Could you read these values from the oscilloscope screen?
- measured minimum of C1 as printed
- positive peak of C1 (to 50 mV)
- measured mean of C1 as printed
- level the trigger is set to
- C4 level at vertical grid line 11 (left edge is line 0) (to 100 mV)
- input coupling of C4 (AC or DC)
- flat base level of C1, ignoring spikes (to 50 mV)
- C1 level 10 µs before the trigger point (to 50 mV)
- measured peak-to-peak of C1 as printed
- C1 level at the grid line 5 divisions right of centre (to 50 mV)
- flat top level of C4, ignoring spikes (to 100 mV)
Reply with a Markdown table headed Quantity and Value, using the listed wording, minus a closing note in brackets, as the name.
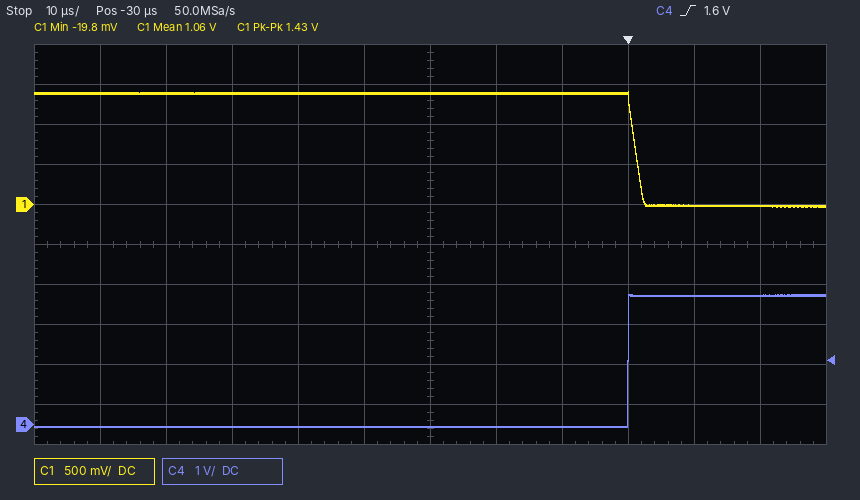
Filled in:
| Quantity | Value |
|---|---|
| measured minimum of C1 as printed | -19.8 mV |
| positive peak of C1 | 1.40 V |
| measured mean of C1 as printed | 1.06 V |
| level the trigger is set to | 1.6 V |
| C4 level at vertical grid line 11 (left edge is line 0) | 3.2 V |
| input coupling of C4 | DC |
| flat base level of C1, ignoring spikes | 0 mV |
| C1 level 10 µs before the trigger point | 1.40 V |
| measured peak-to-peak of C1 as printed | 1.43 V |
| C1 level at the grid line 5 divisions right of centre | 0 mV |
| flat top level of C4, ignoring spikes | 3.2 V |
